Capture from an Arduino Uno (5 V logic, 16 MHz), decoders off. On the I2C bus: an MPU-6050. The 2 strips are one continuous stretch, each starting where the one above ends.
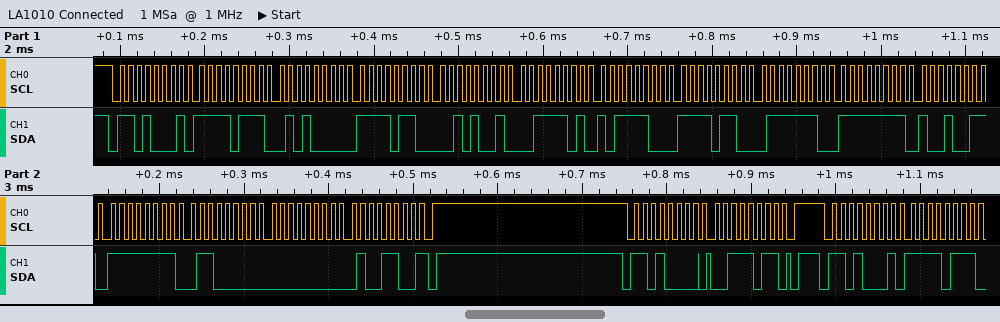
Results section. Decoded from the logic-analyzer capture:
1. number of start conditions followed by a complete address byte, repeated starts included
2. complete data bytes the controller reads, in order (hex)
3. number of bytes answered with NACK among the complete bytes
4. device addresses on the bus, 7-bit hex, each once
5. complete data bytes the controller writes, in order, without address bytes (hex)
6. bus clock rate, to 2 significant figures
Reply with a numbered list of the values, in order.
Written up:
1. 3
2. F7 50 F6 29 3D BC F6 7E FF 93 FF 60 00 4C F7
3. 1
4. 0x68
5. 3B
6. 100 kHz
